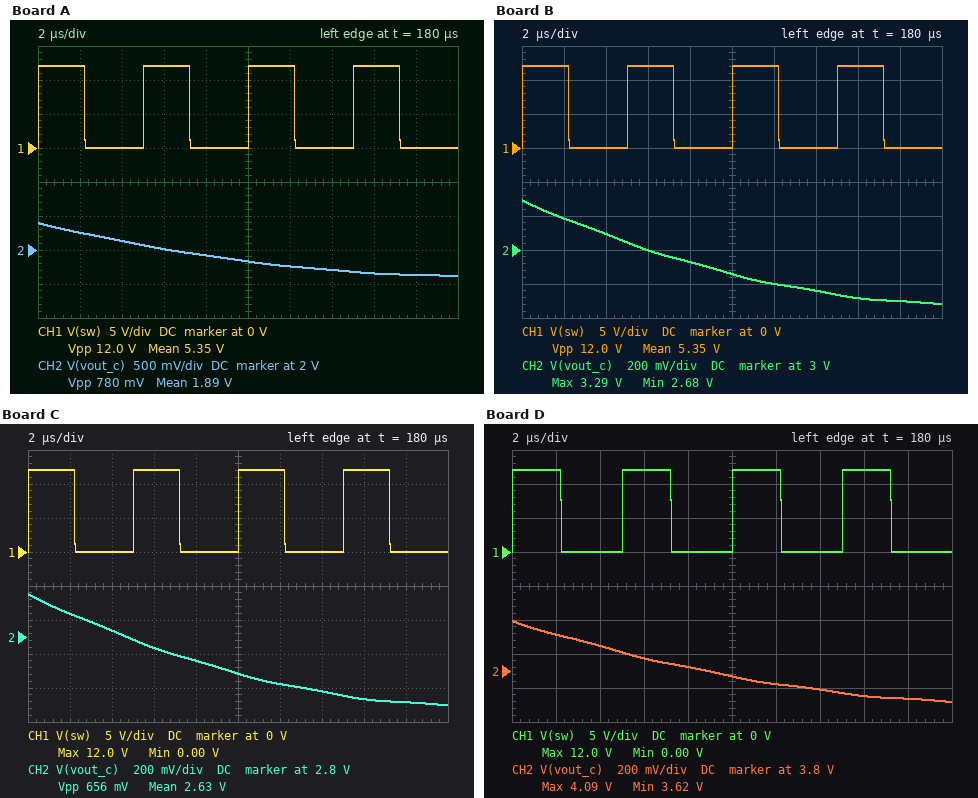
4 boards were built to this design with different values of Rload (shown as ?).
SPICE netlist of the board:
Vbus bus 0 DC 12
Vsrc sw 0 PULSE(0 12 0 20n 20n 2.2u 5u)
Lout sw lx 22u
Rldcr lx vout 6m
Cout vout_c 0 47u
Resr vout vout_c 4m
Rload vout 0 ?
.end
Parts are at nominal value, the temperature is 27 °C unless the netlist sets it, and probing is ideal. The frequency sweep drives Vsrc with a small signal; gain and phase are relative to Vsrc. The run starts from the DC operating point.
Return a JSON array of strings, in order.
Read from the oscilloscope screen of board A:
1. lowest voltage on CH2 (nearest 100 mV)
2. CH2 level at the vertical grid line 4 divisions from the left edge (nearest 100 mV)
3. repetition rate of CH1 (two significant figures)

["1.6 V", "1.9 V", "200 kHz"]
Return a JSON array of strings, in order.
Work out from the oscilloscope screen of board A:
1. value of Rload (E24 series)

["6.8 Ω"]
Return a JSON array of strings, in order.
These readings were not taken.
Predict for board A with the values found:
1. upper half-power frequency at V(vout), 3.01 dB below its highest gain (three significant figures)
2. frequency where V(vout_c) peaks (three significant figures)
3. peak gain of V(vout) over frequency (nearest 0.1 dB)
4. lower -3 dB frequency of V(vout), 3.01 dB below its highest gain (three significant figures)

["5.21 kHz", "4.93 kHz", "18.8 dB", "4.64 kHz"]
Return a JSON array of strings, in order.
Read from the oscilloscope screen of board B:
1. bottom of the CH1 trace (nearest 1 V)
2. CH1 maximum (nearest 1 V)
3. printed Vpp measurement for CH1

["0 V", "12 V", "12.0 V"]
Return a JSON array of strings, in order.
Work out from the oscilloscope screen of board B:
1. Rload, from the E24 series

["3.3 Ω"]
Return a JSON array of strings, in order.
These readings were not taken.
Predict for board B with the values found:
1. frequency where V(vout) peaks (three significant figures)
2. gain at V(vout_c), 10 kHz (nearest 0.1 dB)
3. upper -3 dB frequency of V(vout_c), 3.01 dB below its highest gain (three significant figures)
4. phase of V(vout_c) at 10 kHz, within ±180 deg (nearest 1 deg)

["4.89 kHz", "-9.9 dB", "5.41 kHz", "-172 deg"]
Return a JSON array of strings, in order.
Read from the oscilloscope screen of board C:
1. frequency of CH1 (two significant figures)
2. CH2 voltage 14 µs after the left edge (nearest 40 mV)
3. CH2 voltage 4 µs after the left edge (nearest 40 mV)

["200 kHz", "2.48 V", "2.84 V"]
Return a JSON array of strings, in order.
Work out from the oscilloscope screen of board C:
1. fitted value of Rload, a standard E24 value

["3.9 Ω"]
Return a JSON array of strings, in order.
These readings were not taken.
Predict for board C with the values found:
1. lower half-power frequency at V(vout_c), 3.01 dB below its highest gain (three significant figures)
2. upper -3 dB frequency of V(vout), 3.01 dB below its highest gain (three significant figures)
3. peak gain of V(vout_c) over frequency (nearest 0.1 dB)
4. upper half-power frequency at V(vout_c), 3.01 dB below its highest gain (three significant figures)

["4.41 kHz", "5.36 kHz", "14.5 dB", "5.36 kHz"]
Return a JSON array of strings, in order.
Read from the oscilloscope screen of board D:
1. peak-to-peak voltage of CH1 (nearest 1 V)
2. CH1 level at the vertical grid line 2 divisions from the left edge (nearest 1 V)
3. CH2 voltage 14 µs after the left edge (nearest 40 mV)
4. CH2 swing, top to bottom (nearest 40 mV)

["12 V", "0 V", "3.68 V", "480 mV"]
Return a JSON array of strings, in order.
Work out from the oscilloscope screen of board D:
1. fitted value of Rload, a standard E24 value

["2 Ω"]
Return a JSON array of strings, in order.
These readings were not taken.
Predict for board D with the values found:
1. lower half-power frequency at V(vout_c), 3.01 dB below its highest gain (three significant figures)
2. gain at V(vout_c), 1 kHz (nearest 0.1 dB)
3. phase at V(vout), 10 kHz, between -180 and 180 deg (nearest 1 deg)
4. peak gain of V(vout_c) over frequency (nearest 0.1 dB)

["3.79 kHz", "0.3 dB", "-166 deg", "9.1 dB"]
